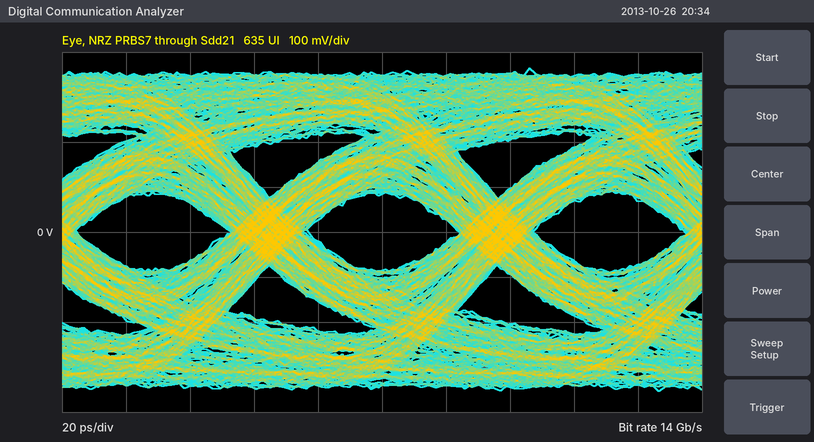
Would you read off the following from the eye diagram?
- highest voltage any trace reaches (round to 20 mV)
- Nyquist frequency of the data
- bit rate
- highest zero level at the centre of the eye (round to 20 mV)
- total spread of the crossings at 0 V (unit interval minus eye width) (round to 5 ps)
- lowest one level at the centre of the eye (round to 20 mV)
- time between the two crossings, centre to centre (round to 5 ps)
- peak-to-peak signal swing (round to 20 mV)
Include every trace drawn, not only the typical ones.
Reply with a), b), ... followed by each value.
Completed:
a) 360 mV
b) 7 GHz
c) 14 Gb/s
d) -80 mV
e) 25 ps
f) 80 mV
g) 70 ps
h) 720 mV
